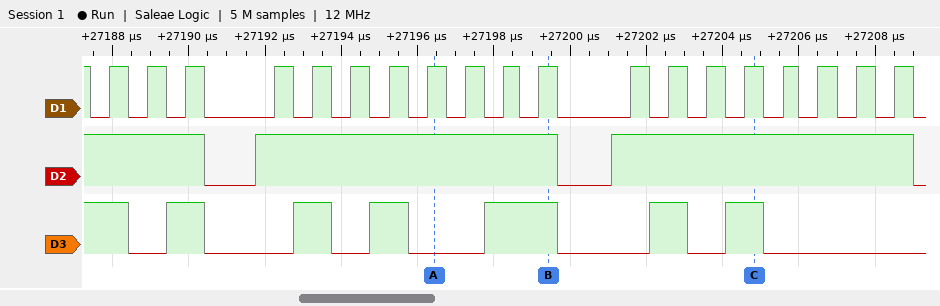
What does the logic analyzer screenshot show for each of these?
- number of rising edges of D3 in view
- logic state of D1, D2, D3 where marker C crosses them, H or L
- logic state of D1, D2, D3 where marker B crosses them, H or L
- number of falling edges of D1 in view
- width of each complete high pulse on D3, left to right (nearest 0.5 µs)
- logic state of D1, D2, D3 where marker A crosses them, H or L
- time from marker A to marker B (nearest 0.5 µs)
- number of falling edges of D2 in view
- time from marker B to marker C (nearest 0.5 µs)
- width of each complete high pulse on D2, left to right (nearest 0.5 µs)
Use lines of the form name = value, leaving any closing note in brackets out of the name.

number of rising edges of D3 in view = 6
logic state of D1, D2, D3 where marker C crosses them, H or L = D1=H, D2=H, D3=H
logic state of D1, D2, D3 where marker B crosses them, H or L = D1=H, D2=H, D3=H
number of falling edges of D1 in view = 20
width of each complete high pulse on D3, left to right = 1 µs, 1 µs, 1 µs, 2 µs, 1 µs, 1 µs
logic state of D1, D2, D3 where marker A crosses them, H or L = D1=H, D2=H, D3=L
time from marker A to marker B = 3 µs
number of falling edges of D2 in view = 3
time from marker B to marker C = 5.5 µs
width of each complete high pulse on D2, left to right = 8 µs, 8 µs
